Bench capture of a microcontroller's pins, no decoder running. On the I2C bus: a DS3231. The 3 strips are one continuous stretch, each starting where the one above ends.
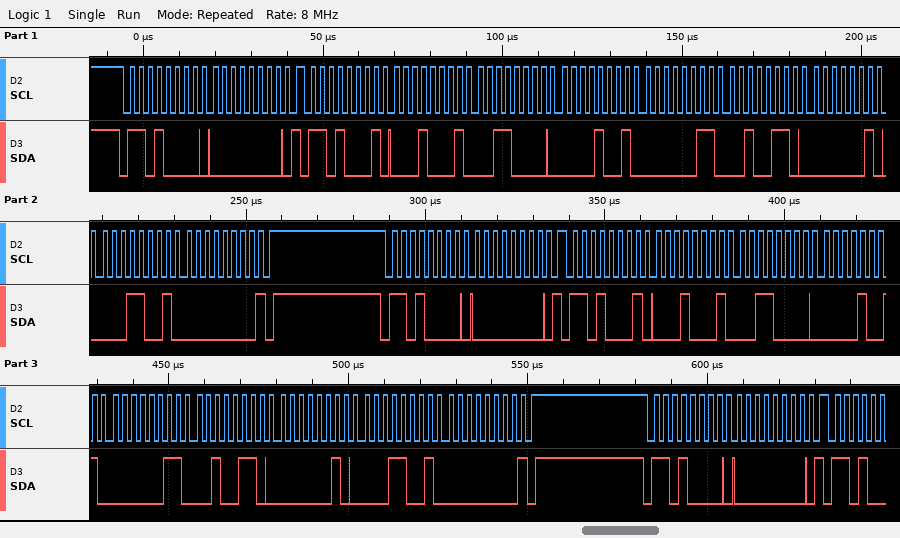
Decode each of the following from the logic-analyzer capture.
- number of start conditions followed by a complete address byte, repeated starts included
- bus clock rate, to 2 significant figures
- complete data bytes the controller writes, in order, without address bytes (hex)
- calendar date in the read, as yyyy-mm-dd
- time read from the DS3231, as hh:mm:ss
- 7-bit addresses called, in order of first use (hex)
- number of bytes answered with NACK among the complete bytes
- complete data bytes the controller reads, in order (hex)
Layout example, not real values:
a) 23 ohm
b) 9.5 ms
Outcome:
a) 5
b) 400 kHz
c) 00 00 00
d) 2019-02-26
e) 09:30:11
f) 0x68
g) 2
h) 11 30 09 03 26 02 19 00 11 30 09 03 26 02 19 00
